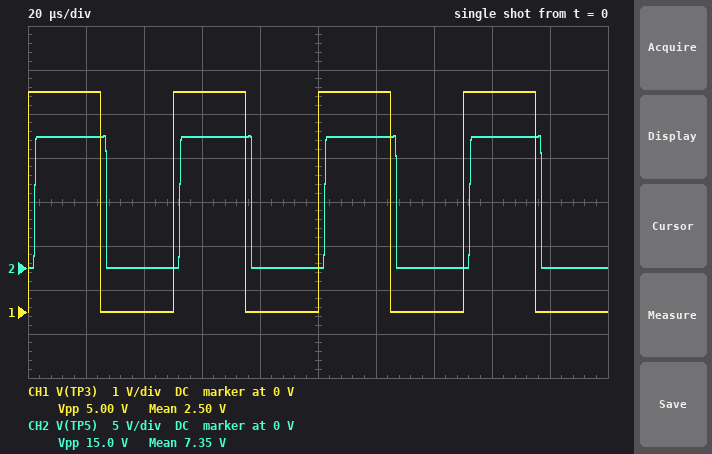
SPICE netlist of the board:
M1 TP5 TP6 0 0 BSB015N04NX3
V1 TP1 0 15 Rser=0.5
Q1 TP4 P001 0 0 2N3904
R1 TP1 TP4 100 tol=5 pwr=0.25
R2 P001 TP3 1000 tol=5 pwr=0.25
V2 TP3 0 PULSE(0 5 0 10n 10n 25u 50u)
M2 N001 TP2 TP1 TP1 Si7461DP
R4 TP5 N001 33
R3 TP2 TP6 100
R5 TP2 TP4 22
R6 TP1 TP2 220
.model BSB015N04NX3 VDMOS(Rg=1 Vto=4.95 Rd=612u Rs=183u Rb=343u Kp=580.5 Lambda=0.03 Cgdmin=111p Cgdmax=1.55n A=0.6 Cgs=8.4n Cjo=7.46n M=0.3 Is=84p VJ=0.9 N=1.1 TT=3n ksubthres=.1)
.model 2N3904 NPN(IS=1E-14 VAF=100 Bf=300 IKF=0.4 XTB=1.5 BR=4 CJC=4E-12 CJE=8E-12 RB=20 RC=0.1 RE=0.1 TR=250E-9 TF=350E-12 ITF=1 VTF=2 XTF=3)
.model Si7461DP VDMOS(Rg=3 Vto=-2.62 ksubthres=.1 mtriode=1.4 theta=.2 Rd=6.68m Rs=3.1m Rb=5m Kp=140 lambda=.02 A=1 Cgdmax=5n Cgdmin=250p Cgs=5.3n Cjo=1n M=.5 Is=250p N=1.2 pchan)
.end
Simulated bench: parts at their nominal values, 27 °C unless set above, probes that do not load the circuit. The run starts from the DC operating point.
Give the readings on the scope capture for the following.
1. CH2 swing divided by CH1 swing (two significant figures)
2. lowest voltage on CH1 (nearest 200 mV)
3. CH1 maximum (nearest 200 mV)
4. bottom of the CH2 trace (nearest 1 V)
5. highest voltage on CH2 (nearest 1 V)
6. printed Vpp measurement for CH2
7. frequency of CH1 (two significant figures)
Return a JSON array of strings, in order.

["3.0", "0 V", "5.0 V", "0 V", "15 V", "15.0 V", "20 kHz"]
